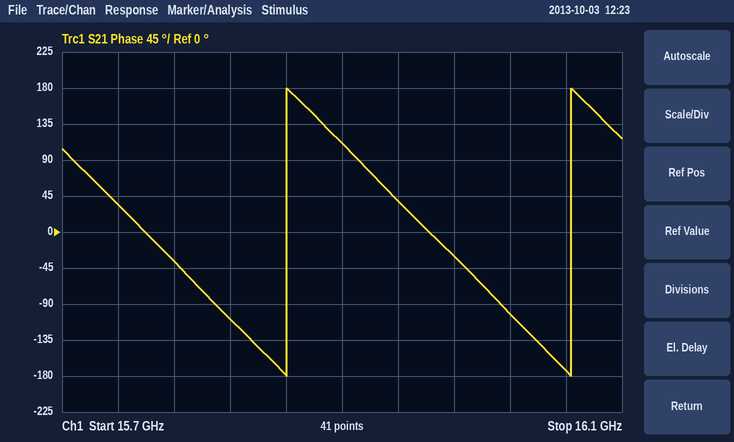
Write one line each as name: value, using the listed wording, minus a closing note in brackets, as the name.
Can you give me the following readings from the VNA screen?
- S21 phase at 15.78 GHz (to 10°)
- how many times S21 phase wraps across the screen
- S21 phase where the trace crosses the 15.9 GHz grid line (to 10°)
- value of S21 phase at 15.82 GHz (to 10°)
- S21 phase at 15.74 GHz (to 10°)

S21 phase at 15.78 GHz: -40°
how many times S21 phase wraps across the screen: 2
S21 phase where the trace crosses the 15.9 GHz grid line: 110°
value of S21 phase at 15.82 GHz: -110°
S21 phase at 15.74 GHz: 30°
